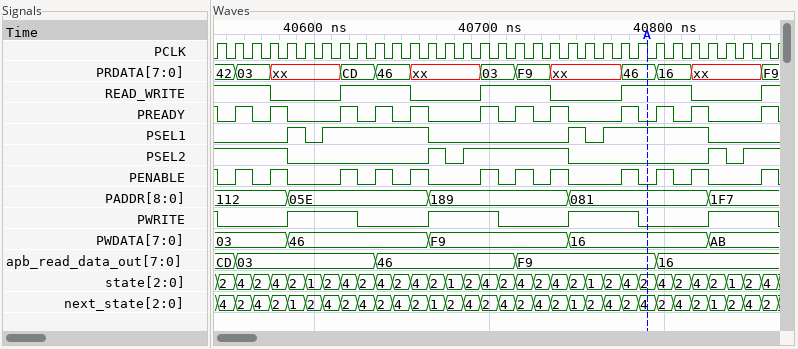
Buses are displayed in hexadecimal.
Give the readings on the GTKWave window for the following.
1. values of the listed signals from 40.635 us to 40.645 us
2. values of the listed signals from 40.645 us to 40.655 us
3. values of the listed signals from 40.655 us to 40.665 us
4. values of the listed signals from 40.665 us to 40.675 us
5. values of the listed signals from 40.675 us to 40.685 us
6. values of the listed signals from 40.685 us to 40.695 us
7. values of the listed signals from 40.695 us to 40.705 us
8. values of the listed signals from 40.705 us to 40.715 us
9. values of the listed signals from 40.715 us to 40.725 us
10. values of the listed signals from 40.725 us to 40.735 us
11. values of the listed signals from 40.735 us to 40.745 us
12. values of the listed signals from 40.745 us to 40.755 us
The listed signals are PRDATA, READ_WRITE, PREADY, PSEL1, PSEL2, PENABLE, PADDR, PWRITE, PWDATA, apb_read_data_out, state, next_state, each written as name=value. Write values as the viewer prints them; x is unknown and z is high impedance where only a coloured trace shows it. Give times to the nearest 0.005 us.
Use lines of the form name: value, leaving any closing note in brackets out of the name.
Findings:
values of the listed signals from 40.635 us to 40.645 us: PRDATA=46, READ_WRITE=1, PREADY=1, PSEL1=1, PSEL2=0, PENABLE=1, PADDR=05E, PWRITE=0, PWDATA=46, apb_read_data_out=46, state=4, next_state=2
values of the listed signals from 40.645 us to 40.655 us: PRDATA=46, READ_WRITE=1, PREADY=0, PSEL1=1, PSEL2=0, PENABLE=0, PADDR=05E, PWRITE=0, PWDATA=46, apb_read_data_out=46, state=2, next_state=4
values of the listed signals from 40.655 us to 40.665 us: PRDATA=xx, READ_WRITE=0, PREADY=1, PSEL1=1, PSEL2=0, PENABLE=1, PADDR=05E, PWRITE=0, PWDATA=46, apb_read_data_out=46, state=4, next_state=2
values of the listed signals from 40.665 us to 40.675 us: PRDATA=xx, READ_WRITE=0, PREADY=0, PSEL1=0, PSEL2=1, PENABLE=0, PADDR=189, PWRITE=1, PWDATA=F9, apb_read_data_out=46, state=2, next_state=1
values of the listed signals from 40.675 us to 40.685 us: PRDATA=xx, READ_WRITE=0, PREADY=0, PSEL1=0, PSEL2=0, PENABLE=0, PADDR=189, PWRITE=1, PWDATA=F9, apb_read_data_out=46, state=1, next_state=2
values of the listed signals from 40.685 us to 40.695 us: PRDATA=xx, READ_WRITE=0, PREADY=0, PSEL1=0, PSEL2=1, PENABLE=0, PADDR=189, PWRITE=1, PWDATA=F9, apb_read_data_out=46, state=2, next_state=4
values of the listed signals from 40.695 us to 40.705 us: PRDATA=03, READ_WRITE=1, PREADY=1, PSEL1=0, PSEL2=1, PENABLE=1, PADDR=189, PWRITE=1, PWDATA=F9, apb_read_data_out=46, state=4, next_state=2
values of the listed signals from 40.705 us to 40.715 us: PRDATA=03, READ_WRITE=1, PREADY=0, PSEL1=0, PSEL2=1, PENABLE=0, PADDR=189, PWRITE=0, PWDATA=F9, apb_read_data_out=46, state=2, next_state=4
values of the listed signals from 40.715 us to 40.725 us: PRDATA=F9, READ_WRITE=1, PREADY=1, PSEL1=0, PSEL2=1, PENABLE=1, PADDR=189, PWRITE=0, PWDATA=F9, apb_read_data_out=F9, state=4, next_state=2
values of the listed signals from 40.725 us to 40.735 us: PRDATA=F9, READ_WRITE=1, PREADY=0, PSEL1=0, PSEL2=1, PENABLE=0, PADDR=189, PWRITE=0, PWDATA=F9, apb_read_data_out=F9, state=2, next_state=4
values of the listed signals from 40.735 us to 40.745 us: PRDATA=xx, READ_WRITE=0, PREADY=1, PSEL1=0, PSEL2=1, PENABLE=1, PADDR=189, PWRITE=0, PWDATA=F9, apb_read_data_out=F9, state=4, next_state=2
values of the listed signals from 40.745 us to 40.755 us: PRDATA=xx, READ_WRITE=0, PREADY=0, PSEL1=1, PSEL2=0, PENABLE=0, PADDR=081, PWRITE=1, PWDATA=16, apb_read_data_out=F9, state=2, next_state=1
